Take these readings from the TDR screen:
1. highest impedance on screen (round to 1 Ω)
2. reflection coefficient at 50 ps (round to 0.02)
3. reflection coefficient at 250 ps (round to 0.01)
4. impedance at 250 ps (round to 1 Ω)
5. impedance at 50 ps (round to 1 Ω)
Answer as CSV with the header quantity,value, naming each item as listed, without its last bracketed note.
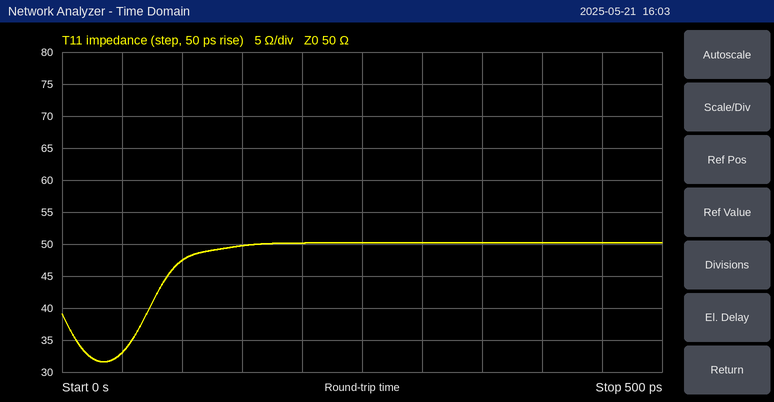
quantity,value
highest impedance on screen,50 Ω
reflection coefficient at 50 ps,-0.20
reflection coefficient at 250 ps,0.00
impedance at 250 ps,50 Ω
impedance at 50 ps,33 Ω
